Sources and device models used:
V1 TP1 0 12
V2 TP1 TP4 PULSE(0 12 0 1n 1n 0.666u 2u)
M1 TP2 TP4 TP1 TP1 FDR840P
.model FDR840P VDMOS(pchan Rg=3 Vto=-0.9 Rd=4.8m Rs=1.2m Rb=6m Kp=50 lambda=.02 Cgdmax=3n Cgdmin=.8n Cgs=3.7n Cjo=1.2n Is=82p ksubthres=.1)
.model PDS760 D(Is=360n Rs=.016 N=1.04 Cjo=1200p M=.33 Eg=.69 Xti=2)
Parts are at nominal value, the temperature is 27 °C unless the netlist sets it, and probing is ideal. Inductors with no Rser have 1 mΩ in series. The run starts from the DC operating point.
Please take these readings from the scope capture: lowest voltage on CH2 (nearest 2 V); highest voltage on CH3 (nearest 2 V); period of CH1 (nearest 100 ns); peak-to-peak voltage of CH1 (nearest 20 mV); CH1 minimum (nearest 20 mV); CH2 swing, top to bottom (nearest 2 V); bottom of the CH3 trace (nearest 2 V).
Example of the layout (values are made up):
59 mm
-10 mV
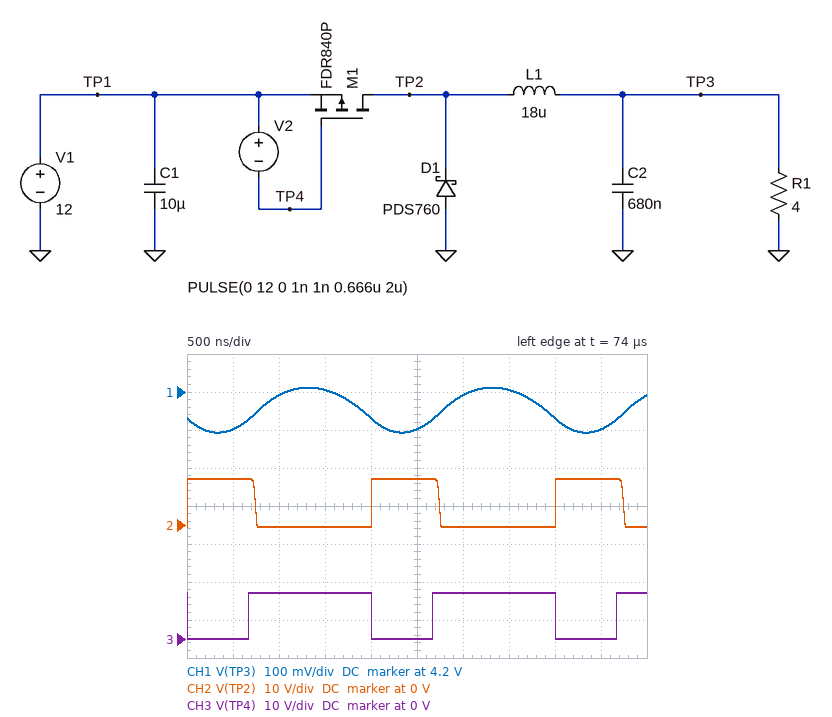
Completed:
0 V
12 V
2.0 µs
120 mV
4.10 V
12 V
0 V
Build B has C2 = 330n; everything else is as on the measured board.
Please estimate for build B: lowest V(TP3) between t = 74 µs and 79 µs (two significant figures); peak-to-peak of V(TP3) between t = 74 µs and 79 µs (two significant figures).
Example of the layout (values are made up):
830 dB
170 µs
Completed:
4.0 V
240 mV
